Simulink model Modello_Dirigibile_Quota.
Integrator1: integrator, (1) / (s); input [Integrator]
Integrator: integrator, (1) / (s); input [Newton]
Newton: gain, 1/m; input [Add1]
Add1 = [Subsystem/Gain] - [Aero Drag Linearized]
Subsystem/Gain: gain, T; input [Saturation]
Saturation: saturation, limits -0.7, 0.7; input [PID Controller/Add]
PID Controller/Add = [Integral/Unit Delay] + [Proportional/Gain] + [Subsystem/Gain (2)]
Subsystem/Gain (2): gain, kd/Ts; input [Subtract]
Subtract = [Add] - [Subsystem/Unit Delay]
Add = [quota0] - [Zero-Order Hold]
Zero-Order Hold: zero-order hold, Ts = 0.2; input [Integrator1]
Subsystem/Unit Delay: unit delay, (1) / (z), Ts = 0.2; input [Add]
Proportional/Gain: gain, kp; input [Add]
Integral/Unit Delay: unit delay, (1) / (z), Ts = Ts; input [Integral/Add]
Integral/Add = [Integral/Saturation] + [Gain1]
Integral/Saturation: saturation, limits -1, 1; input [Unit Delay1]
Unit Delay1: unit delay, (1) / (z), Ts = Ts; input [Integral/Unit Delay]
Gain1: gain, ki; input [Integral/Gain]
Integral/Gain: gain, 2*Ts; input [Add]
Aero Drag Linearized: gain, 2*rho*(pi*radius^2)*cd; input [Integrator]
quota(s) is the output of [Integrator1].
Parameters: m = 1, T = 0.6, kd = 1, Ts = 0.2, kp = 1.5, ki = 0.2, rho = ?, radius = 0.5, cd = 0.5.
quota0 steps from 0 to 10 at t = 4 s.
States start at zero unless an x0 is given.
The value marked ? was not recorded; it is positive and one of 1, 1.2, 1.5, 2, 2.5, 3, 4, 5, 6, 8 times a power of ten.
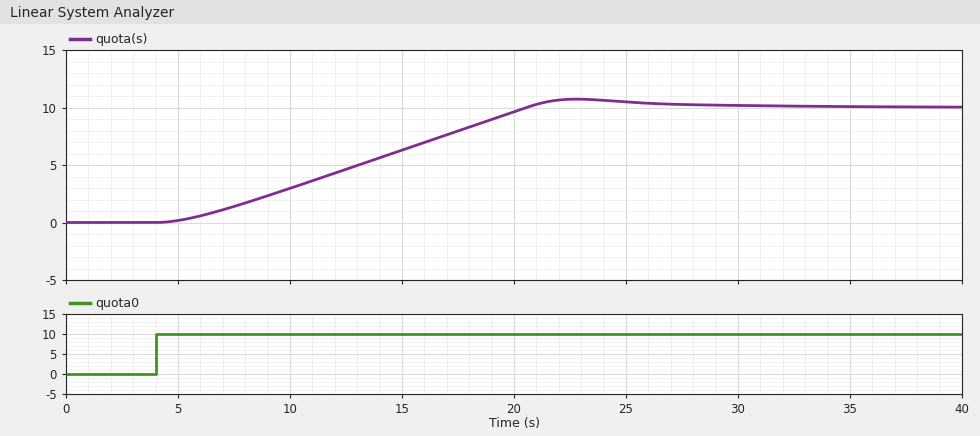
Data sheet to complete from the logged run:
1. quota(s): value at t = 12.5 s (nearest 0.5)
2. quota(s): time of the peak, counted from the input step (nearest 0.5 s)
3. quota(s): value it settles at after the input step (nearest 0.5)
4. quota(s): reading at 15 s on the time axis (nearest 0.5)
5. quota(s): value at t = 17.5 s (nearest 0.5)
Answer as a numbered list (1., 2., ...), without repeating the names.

1. 4.5
2. 19.0 s
3. 10.0
4. 6.5
5. 8.0
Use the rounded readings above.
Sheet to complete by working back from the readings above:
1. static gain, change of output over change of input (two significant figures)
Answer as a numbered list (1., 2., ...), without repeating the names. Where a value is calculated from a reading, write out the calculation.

1. (10 - 0) / (10 - 0) = 1.0
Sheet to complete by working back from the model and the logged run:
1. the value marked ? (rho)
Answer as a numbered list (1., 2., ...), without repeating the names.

1. 0.8
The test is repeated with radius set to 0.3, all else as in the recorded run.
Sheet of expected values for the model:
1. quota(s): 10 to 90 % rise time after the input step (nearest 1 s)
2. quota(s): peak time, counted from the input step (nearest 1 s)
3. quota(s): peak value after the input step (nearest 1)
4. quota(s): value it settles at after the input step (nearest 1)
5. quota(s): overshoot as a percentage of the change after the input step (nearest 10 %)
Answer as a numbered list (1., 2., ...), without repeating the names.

1. 6 s
2. 12 s
3. 12
4. 10
5. 20 %
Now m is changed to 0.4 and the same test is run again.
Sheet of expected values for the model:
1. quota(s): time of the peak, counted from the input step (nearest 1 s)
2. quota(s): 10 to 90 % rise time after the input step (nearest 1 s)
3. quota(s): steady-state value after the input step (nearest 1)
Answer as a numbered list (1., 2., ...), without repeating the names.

1. 18 s
2. 12 s
3. 10
